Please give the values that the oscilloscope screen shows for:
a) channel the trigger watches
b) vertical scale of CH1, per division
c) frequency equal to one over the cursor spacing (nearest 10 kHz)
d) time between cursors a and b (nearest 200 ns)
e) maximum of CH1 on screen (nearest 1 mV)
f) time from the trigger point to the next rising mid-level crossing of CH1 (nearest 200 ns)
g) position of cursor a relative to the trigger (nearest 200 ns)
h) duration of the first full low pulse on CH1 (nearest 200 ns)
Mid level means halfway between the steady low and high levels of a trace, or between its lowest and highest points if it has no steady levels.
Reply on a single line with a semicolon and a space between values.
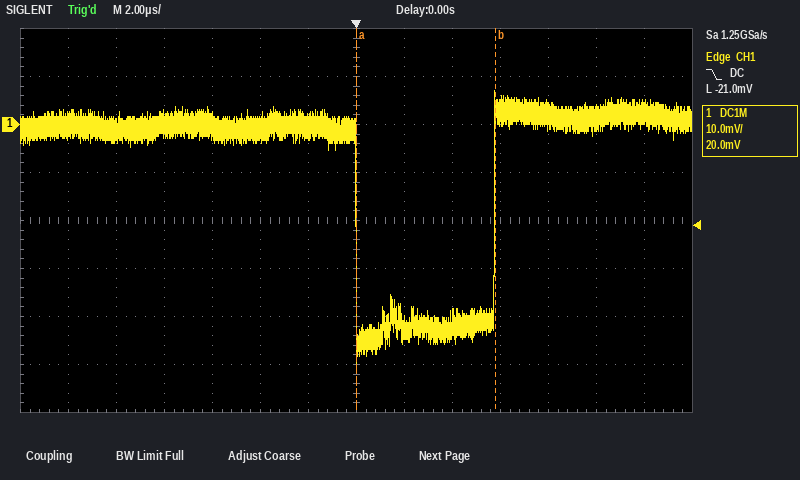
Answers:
CH1; 10 mV; 170 kHz; 5.8 µs; 7 mV; 5.8 µs; 0.0 µs; 5.8 µs
